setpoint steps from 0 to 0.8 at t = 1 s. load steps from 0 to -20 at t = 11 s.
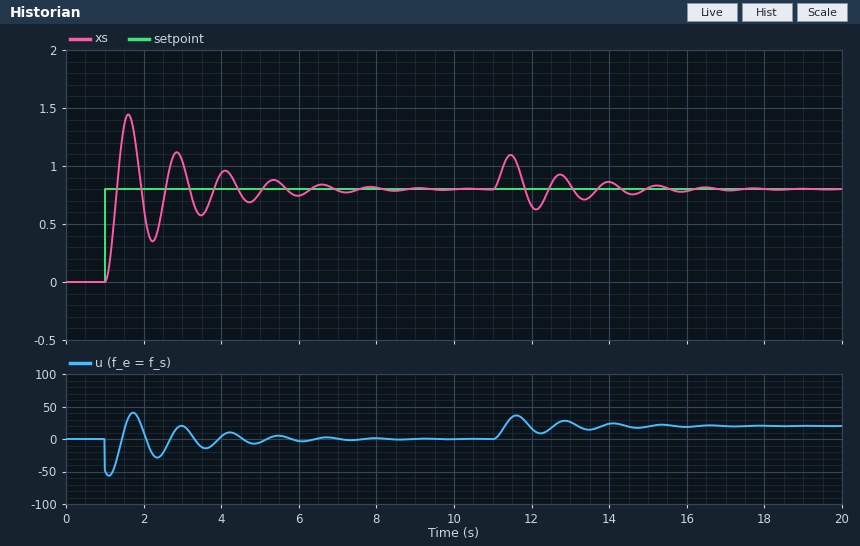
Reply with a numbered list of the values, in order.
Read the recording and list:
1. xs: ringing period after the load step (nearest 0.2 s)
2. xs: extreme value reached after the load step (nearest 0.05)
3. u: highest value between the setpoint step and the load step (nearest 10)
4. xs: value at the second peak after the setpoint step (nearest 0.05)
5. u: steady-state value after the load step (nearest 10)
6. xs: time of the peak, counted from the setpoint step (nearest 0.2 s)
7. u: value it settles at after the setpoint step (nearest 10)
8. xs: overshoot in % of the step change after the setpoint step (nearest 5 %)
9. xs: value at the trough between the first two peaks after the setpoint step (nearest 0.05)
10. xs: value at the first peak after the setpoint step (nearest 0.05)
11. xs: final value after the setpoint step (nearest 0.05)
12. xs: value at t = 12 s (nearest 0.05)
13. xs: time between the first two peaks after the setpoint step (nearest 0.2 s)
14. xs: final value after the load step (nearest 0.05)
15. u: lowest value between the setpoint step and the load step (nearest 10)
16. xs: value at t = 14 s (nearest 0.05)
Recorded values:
1. 1.2 s
2. 1.10
3. 40
4. 1.10
5. 20
6. 0.6 s
7. 0
8. 80 %
9. 0.35
10. 1.45
11. 0.80
12. 0.65
13. 1.2 s
14. 0.80
15. -60
16. 0.85
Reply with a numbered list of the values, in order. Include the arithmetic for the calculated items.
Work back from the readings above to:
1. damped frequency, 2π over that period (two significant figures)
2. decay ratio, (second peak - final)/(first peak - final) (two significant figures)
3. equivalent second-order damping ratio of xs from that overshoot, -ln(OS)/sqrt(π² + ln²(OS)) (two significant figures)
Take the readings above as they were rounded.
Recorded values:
1. 2π / 1.2 = 5.2 rad/s
2. (1.1 - 0.8) / (1.45 - 0.8) = 0.46
3. ln(0.8) = -0.223; 0.223 / sqrt(9.870 + 0.050) = 0.071
